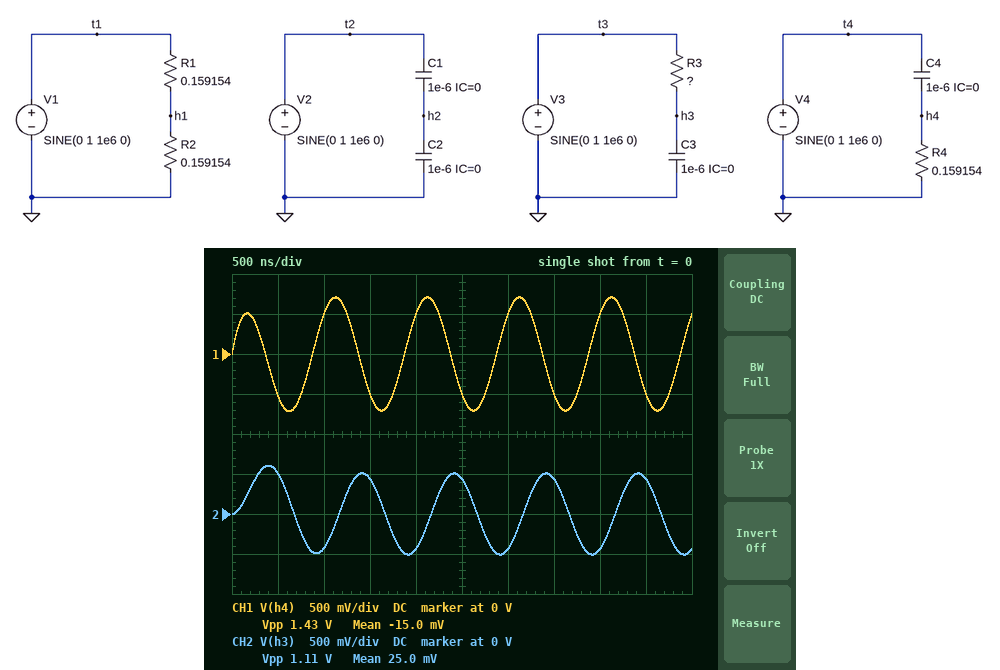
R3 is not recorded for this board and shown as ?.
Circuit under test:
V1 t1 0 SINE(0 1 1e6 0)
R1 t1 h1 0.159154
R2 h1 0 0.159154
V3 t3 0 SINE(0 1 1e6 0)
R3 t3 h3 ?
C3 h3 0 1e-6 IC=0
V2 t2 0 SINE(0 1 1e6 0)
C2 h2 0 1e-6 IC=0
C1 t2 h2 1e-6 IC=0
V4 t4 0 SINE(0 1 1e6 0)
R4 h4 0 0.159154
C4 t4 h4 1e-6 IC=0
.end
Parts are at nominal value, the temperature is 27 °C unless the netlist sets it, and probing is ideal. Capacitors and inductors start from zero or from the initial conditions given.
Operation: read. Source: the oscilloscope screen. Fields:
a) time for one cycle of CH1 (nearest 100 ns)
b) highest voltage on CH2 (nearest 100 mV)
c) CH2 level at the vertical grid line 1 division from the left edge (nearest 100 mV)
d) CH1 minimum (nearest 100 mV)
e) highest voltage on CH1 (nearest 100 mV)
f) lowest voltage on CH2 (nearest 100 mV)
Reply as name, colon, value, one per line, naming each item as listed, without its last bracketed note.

time for one cycle of CH1: 1.0 µs
highest voltage on CH2: 600 mV
CH2 level at the vertical grid line 1 division from the left edge: 500 mV
CH1 minimum: -700 mV
highest voltage on CH1: 700 mV
lowest voltage on CH2: -500 mV
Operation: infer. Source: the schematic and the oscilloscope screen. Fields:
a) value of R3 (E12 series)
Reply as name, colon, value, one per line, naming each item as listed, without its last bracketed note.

value of R3: 0.27 Ω
